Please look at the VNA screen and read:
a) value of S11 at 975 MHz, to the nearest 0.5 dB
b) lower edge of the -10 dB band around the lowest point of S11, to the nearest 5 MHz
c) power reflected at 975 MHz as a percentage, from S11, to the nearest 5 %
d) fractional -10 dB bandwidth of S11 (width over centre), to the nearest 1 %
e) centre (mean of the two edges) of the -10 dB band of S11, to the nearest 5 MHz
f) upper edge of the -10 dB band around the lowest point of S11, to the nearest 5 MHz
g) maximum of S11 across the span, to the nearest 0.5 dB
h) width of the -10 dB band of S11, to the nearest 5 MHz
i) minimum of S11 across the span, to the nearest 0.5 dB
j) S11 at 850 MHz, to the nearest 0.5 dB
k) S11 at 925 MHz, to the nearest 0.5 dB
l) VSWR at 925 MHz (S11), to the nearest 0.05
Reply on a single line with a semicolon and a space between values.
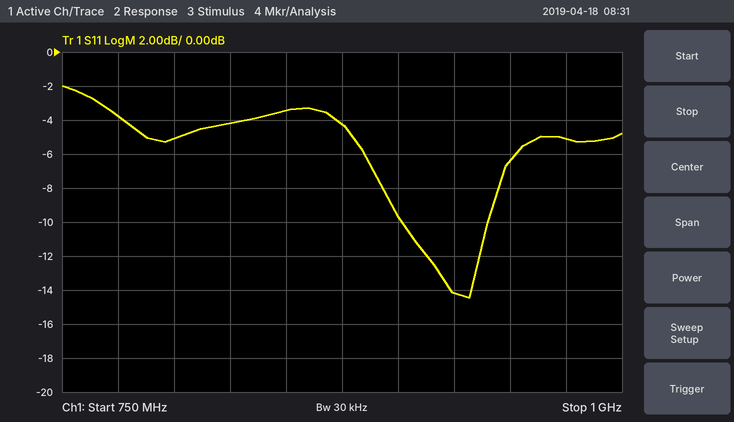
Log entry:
-5.0 dB; 900 MHz; 30 %; 4 %; 920 MHz; 940 MHz; -2.0 dB; 40 MHz; -14.5 dB; -3.5 dB; -14.0 dB; 1.50
